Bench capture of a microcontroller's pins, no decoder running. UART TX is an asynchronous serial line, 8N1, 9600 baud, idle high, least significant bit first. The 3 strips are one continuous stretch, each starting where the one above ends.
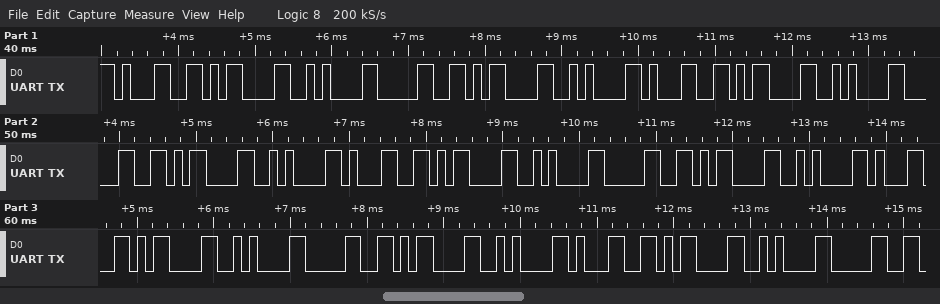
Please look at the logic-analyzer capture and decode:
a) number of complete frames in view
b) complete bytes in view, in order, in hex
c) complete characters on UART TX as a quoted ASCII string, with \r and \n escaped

28
0x31 0x0D 0x0A 0x30 0x0D 0x0A 0x31 0x0D 0x0A 0x30 0x0D 0x0A 0x31 0x0D 0x0A 0x30 0x0D 0x0A 0x31 0x0D 0x0A 0x30 0x0D 0x0A 0x31 0x0D 0x0A 0x30
"1\r\n0\r\n1\r\n0\r\n1\r\n0\r\n1\r\n0\r\n1\r\n0"
